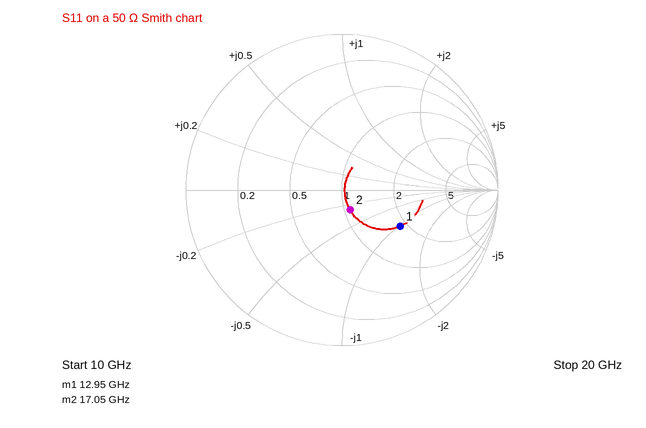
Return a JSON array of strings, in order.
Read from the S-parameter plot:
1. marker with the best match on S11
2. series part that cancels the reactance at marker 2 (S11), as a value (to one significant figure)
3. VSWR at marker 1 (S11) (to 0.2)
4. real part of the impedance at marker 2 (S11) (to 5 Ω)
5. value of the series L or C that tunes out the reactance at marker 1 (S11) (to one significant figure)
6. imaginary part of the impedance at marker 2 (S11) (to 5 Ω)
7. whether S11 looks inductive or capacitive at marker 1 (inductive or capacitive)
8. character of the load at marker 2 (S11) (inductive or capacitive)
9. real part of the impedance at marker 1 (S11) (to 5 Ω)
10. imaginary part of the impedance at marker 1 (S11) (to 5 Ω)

["marker 2", "100 pH", "2.6", "55 Ω", "600 pH", "-15 Ω", "capacitive", "capacitive", "90 Ω", "-50 Ω"]
